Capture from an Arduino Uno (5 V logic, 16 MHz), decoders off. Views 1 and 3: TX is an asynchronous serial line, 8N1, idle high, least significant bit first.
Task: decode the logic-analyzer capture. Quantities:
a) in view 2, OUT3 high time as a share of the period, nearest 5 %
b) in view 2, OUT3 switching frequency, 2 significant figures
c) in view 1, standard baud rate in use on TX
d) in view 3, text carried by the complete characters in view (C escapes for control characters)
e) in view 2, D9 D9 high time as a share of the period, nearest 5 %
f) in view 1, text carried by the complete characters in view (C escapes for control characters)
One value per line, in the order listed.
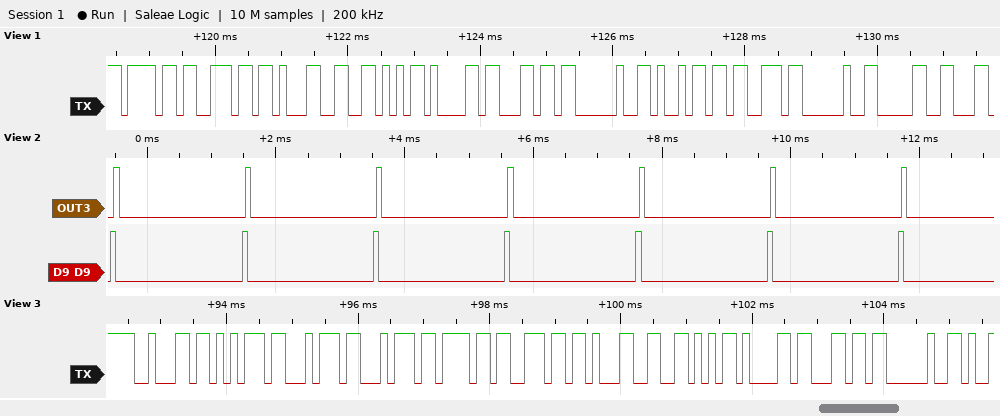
5 %
490 Hz
9600 baud
"button1Val "
5 %
"on1Val is 0"
